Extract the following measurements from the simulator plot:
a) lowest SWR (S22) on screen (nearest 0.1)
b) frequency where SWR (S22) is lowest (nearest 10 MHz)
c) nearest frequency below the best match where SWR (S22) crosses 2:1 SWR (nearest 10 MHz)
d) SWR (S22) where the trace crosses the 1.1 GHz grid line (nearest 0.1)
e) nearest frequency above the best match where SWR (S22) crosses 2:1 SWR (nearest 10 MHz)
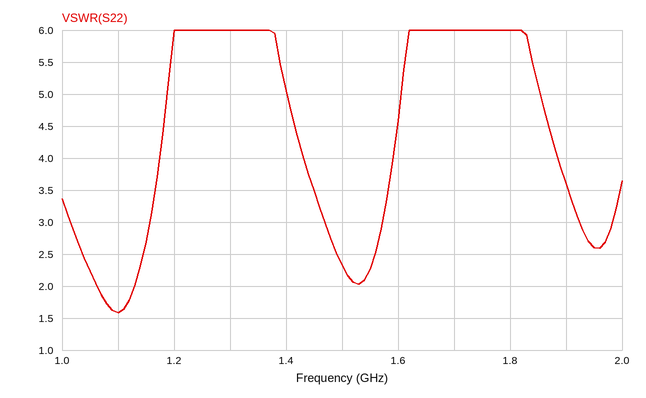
1.6
1.10 GHz
1.06 GHz
1.6
1.13 GHz
